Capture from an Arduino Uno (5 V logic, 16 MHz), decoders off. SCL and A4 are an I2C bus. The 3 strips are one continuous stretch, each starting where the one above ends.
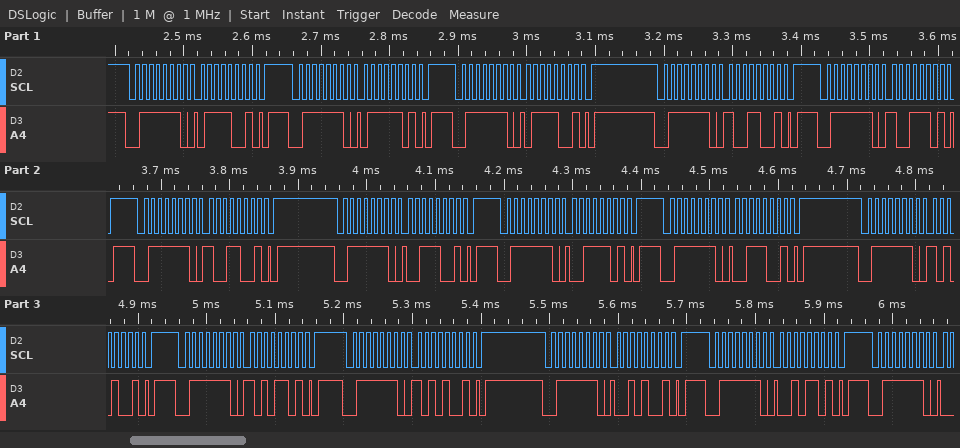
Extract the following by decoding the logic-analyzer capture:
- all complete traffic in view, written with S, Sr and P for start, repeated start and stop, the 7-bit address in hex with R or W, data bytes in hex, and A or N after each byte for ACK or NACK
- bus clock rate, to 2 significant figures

S 3FW A 79 A P S 3FW A 7D A P S 3FW A 79 A P S 3FW A 99 A P S 3FW A 9D A P S 3FW A 99 A P S 3FW A 39 A P S 3FW A 3D A P S 3FW A 39 A P S 3FW A A9 A P S 3FW A AD A P S 3FW A A9 A P S 3FW A 29 A P S 3FW A 2D A P S 3FW A
100 kHz
